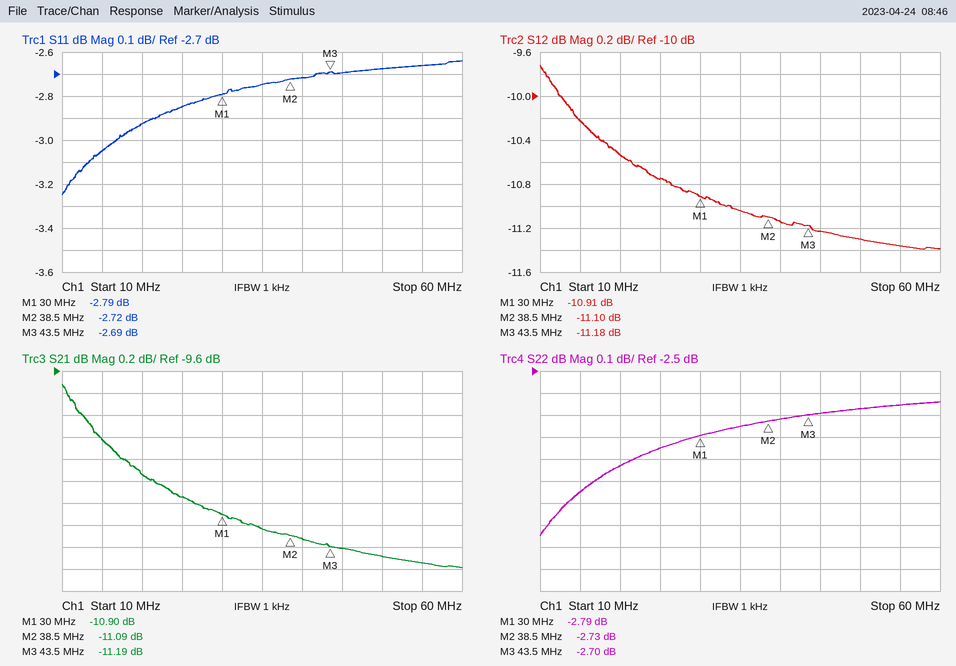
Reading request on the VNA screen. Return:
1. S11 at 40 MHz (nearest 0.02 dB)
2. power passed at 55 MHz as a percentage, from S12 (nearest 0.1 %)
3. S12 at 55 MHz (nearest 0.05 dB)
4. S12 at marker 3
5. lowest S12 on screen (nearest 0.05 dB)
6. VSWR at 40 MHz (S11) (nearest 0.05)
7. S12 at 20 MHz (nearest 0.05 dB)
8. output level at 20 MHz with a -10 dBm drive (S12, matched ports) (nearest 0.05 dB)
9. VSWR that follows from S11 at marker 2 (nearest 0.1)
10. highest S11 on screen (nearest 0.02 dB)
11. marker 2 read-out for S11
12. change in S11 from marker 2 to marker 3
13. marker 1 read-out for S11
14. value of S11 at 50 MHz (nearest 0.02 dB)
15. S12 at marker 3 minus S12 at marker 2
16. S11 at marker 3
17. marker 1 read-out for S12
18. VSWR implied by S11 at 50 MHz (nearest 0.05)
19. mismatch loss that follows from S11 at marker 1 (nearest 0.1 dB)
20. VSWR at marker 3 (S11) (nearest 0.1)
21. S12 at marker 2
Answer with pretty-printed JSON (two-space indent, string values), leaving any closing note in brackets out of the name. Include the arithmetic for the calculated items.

{
  "S11 at 40 MHz": "-2.72 dB",
  "power passed at 55 MHz as a percentage, from S12": "10^(-11.35/10) ≈ 7.3 %",
  "S12 at 55 MHz": "-11.35 dB",
  "S12 at marker 3": "-11.18 dB",
  "lowest S12 on screen": "-11.40 dB",
  "VSWR at 40 MHz (S11)": "|Γ| = 10^(-2.72/20) = 0.7311; VSWR = (1 + 0.7311)/(1 − 0.7311) ≈ 6.44, so 6.45 to the nearest 0.05",
  "S12 at 20 MHz": "-10.55 dB",
  "output level at 20 MHz with a -10 dBm drive (S12, matched ports)": "-10 dBm + (-10.55 dB) = -20.55 dBm",
  "VSWR that follows from S11 at marker 2": "(1 + 0.7311)/(1 − 0.7311) ≈ 6.4",
  "highest S11 on screen": "-2.64 dB",
  "marker 2 read-out for S11": "-2.72 dB",
  "change in S11 from marker 2 to marker 3": "-2.69 − (-2.72) = 0.03 dB",
  "marker 1 read-out for S11": "-2.79 dB",
  "value of S11 at 50 MHz": "-2.68 dB",
  "S12 at marker 3 minus S12 at marker 2": "-11.18 − (-11.1) = -0.08 dB",
  "S11 at marker 3": "-2.69 dB",
  "marker 1 read-out for S12": "-10.91 dB",
  "VSWR implied by S11 at 50 MHz": "|Γ| = 10^(-2.68/20) = 0.7345; VSWR = (1 + 0.7345)/(1 − 0.7345) ≈ 6.53, so 6.55 to the nearest 0.05",
  "mismatch loss that follows from S11 at marker 1": "−10 log10(1 − 10^(-2.79/10)) ≈ 3.2 dB",
  "VSWR at marker 3 (S11)": "(1 + 0.7337)/(1 − 0.7337) ≈ 6.5",
  "S12 at marker 2": "-11.10 dB"
}
